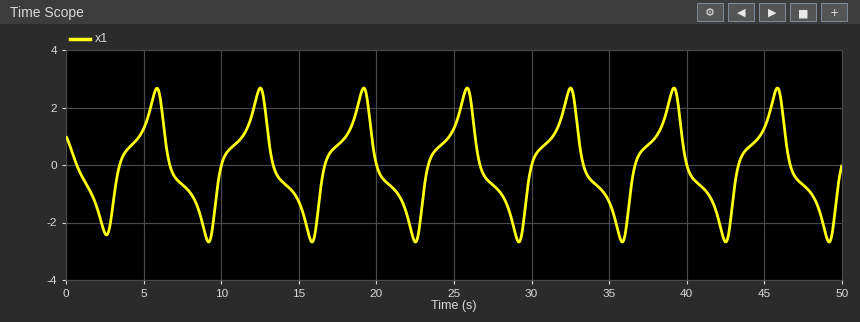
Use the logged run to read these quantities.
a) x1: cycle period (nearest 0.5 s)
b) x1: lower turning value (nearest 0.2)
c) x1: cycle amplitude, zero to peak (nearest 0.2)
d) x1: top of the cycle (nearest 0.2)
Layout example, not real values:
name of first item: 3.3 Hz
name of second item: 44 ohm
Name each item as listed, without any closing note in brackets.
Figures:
x1: cycle period: 6.5 s
x1: lower turning value: -2.6
x1: cycle amplitude, zero to peak: 2.6
x1: top of the cycle: 2.6
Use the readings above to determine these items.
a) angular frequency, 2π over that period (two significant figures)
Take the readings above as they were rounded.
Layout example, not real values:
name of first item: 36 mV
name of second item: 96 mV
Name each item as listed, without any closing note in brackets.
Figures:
angular frequency, 2π over that period: 0.97 rad/s
